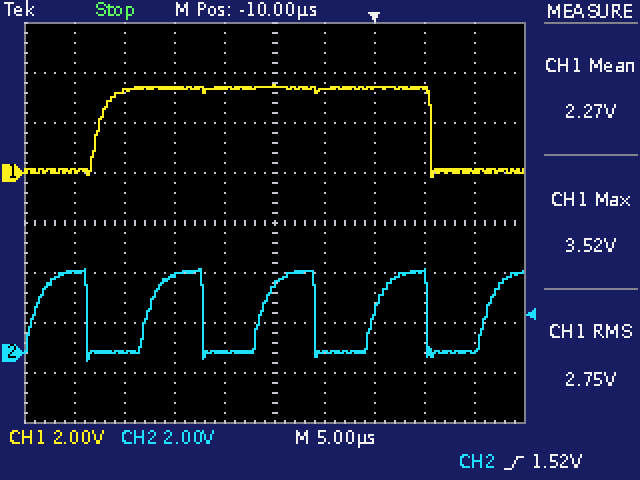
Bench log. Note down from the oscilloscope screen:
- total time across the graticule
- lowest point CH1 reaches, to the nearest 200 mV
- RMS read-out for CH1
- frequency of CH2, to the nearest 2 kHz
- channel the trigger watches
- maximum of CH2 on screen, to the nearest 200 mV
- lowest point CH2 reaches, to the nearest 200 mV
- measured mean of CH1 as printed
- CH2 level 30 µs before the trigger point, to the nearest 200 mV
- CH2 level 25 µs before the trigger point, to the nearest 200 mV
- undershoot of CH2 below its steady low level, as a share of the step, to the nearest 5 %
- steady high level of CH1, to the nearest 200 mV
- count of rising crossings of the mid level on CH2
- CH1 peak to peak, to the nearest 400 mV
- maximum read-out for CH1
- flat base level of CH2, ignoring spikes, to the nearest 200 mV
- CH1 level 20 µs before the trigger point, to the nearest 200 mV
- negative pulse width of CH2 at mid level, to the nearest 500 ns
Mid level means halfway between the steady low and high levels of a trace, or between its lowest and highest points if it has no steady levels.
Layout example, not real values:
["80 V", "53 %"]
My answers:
["50 µs", "-200 mV", "2.75 V", "88 kHz", "CH2", "3.4 V", "-400 mV", "2.27 V", "3.2 V", "0.0 V", "10 %", "3.4 V", "5", "3.6 V", "3.52 V", "0.0 V", "3.4 V", "6.0 µs"]
